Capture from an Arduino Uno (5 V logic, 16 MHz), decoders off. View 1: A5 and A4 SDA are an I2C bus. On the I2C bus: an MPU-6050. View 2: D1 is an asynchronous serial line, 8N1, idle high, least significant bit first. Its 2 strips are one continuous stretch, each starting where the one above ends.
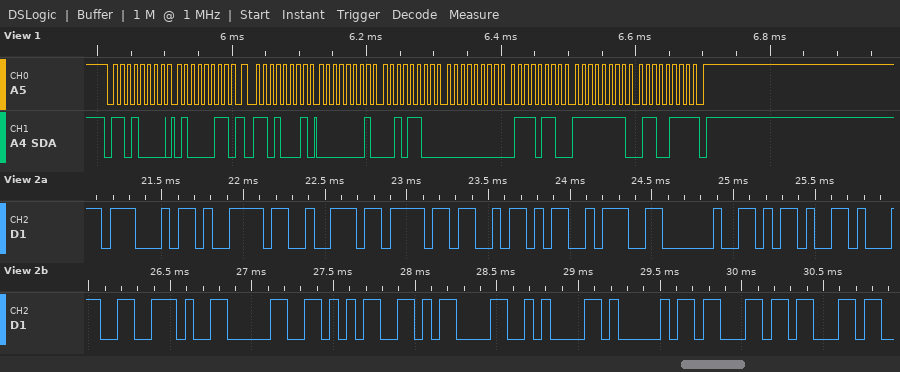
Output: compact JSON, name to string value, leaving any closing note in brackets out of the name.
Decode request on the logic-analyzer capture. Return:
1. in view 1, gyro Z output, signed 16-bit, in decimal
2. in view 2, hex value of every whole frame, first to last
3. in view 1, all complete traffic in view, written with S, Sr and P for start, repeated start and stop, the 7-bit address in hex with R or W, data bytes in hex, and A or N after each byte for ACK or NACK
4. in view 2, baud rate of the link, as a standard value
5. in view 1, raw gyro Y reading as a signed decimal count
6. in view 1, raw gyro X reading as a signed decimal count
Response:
{"in view 1, gyro Z output, signed 16-bit, in decimal": "-153", "in view 2, hex value of every whole frame, first to last": "47 79 72 6F 5A 3A 20 2D 31 2E 30 35 0D 0A 41 63 63", "in view 1, all complete traffic in view, written with S, Sr and P for start, repeated start and stop, the 7-bit address in hex with R or W, data bytes in hex, and A or N after each byte for ACK or NACK": "S 68W A 43 A Sr 68R A 01 A 2C A 00 A 76 A FF A 67 N P", "in view 2, baud rate of the link, as a standard value": "19200 baud", "in view 1, raw gyro Y reading as a signed decimal count": "118", "in view 1, raw gyro X reading as a signed decimal count": "300"}
